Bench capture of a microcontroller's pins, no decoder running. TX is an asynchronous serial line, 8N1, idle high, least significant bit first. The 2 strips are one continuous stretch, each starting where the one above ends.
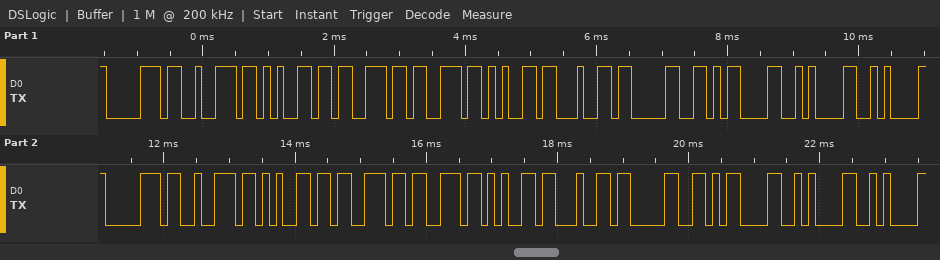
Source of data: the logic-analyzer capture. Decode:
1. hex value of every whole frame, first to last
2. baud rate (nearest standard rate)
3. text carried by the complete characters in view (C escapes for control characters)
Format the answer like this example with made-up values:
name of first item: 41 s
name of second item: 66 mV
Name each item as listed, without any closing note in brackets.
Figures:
hex value of every whole frame, first to last: 70 72 65 73 73 65 64 30 0D 0A 0A 70 72 65 73 73 65 64 30 0D 0A 0A
baud rate: 9600 baud
text carried by the complete characters in view: "pressed0\r\n\npressed0\r\n\n"
